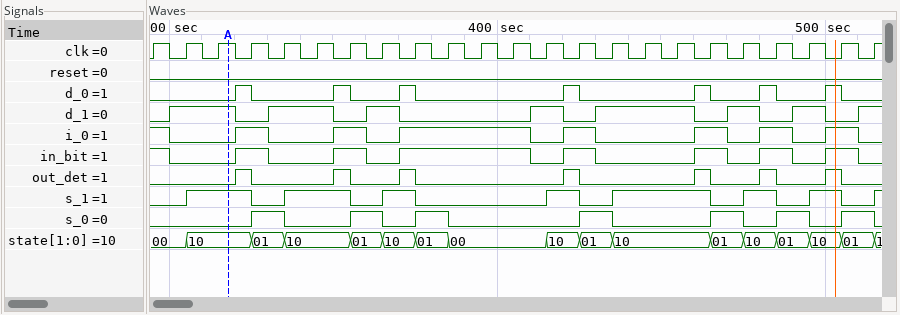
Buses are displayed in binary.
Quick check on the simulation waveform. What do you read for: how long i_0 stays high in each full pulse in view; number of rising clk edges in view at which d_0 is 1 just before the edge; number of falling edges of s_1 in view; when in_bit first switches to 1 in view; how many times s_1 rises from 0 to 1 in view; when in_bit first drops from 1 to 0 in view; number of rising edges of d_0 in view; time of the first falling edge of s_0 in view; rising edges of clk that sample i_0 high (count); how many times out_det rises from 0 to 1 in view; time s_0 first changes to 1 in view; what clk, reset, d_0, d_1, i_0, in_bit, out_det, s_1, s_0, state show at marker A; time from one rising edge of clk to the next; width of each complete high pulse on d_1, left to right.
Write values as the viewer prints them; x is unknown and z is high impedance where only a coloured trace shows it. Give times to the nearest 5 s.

10 s, 10 s, 40 s, 10 s, 10 s, 10 s, 10 s
7
7
320 s
8
300 s
7
335 s
11
7
325 s
clk=1, reset=0, d_0=0, d_1=1, i_0=0, in_bit=0, out_det=0, s_1=1, s_0=0, state=10
10 s
20 s, 20 s, 10 s, 10 s, 30 s, 10 s, 10 s
